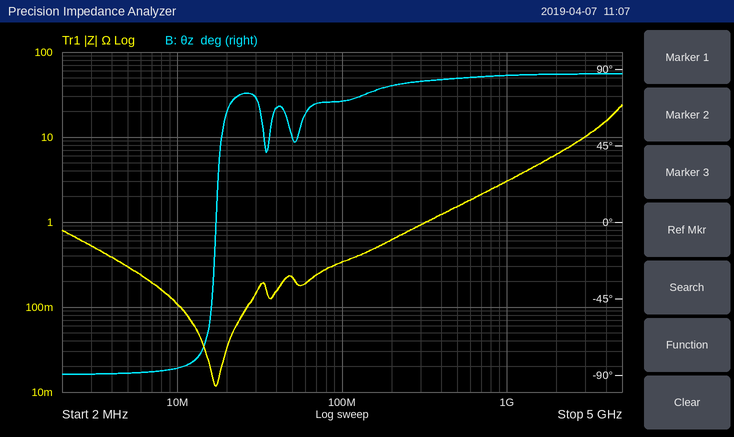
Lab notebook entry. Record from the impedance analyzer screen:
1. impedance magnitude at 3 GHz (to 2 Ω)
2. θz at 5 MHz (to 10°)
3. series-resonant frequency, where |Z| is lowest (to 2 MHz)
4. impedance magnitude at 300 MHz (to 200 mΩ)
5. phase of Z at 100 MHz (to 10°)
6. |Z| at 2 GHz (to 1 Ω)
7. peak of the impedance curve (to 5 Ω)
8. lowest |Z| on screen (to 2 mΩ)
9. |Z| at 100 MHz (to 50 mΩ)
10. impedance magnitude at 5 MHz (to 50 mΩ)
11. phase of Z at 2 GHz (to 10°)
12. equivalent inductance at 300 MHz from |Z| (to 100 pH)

10 Ω
-90°
18 MHz
1.0 Ω
70°
6 Ω
25 Ω
12 mΩ
350 mΩ
300 mΩ
90°
500 pH
